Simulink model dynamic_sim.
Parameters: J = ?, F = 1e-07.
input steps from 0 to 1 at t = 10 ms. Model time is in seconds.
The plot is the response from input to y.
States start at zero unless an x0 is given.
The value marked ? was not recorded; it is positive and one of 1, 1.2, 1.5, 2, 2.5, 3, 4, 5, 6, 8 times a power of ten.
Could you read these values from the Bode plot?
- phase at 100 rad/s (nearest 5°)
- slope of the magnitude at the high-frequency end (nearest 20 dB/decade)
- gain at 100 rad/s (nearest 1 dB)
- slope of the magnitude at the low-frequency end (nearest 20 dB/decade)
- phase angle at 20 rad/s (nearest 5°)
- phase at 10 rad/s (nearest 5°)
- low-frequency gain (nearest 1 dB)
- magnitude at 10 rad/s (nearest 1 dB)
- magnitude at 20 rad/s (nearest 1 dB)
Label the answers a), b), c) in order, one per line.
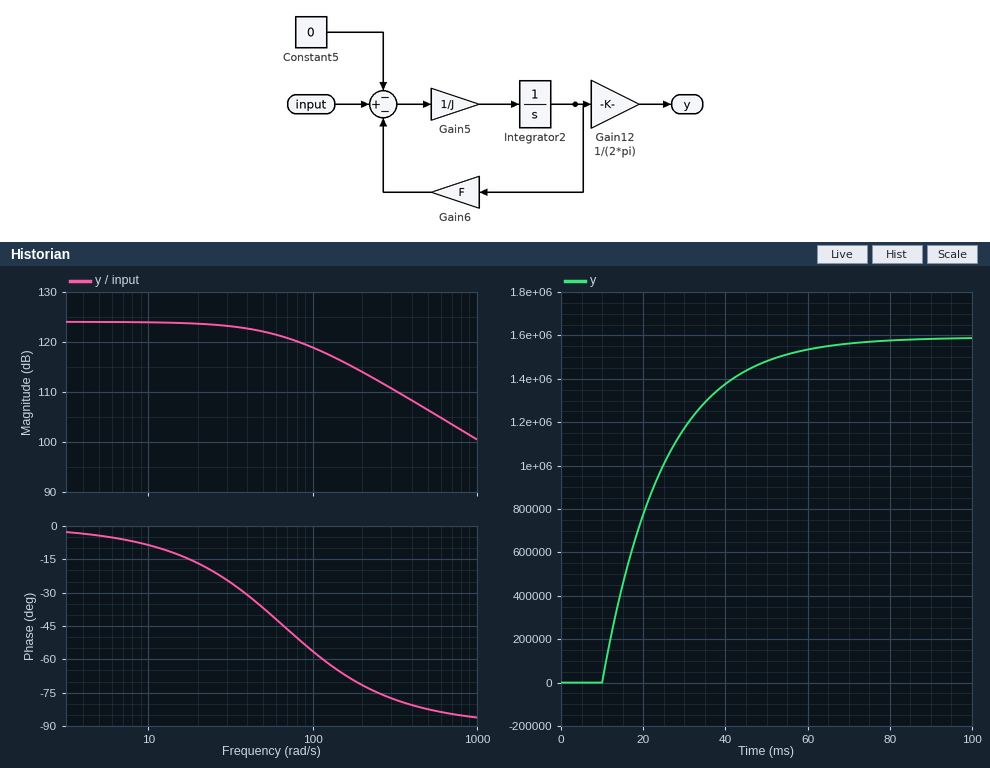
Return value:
a) -55°
b) -20 dB/decade
c) 119 dB
d) 0 dB/decade
e) -15°
f) -10°
g) 124 dB
h) 124 dB
i) 124 dB
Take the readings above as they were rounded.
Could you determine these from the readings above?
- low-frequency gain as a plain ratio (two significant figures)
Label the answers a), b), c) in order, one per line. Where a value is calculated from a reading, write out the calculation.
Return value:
a) 10^(124 / 20) = 1600000
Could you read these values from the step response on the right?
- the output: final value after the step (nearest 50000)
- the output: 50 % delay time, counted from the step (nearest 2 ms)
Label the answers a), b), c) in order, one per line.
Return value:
a) 1600000
b) 10 ms
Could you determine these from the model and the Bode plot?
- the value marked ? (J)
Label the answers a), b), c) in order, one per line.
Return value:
a) 1.5e-09
